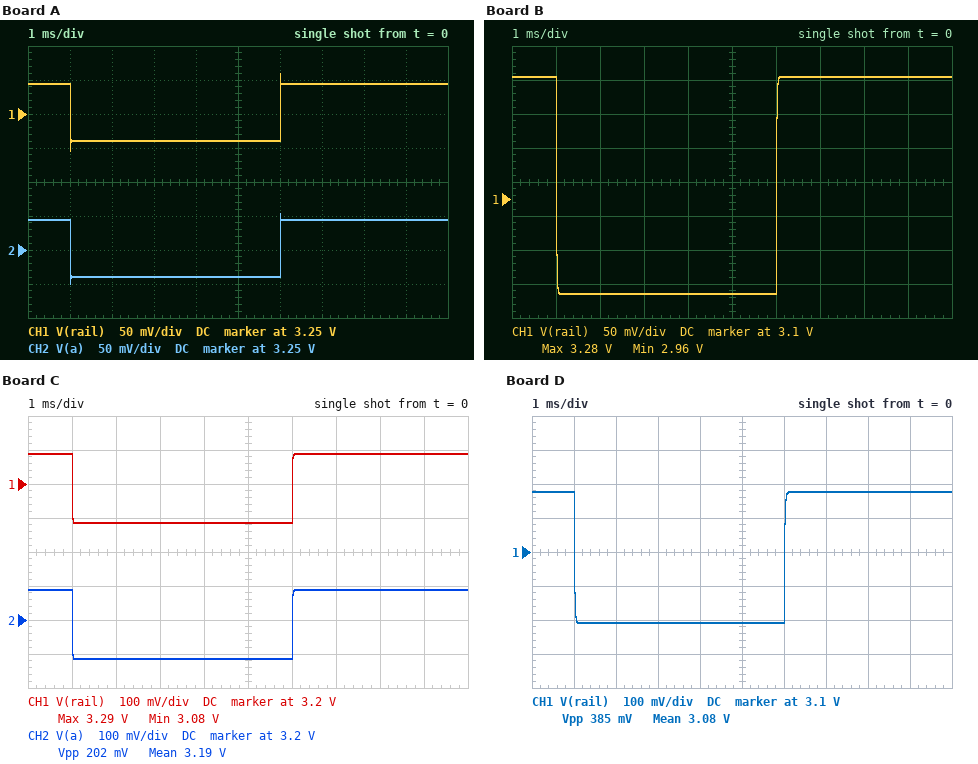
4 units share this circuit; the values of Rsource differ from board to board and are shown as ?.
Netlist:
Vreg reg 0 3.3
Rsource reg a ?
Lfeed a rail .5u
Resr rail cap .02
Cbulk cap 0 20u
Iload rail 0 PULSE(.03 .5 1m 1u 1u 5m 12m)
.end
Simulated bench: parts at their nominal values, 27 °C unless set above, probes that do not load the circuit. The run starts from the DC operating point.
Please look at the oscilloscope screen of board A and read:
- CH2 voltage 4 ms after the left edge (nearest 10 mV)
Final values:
3.21 V
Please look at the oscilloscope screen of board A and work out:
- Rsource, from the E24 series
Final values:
0.18 Ω
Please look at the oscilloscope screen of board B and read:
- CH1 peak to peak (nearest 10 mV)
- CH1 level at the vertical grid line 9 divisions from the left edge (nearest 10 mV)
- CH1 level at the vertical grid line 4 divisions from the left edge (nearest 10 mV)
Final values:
320 mV
3.28 V
2.96 V
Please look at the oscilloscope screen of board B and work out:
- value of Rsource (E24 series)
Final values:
0.68 Ω
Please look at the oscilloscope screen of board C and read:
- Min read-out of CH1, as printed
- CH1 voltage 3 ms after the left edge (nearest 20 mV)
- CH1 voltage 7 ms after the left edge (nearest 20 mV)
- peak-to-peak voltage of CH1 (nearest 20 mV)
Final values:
3.08 V
3.08 V
3.28 V
200 mV
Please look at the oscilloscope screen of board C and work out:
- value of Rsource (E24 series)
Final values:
0.43 Ω
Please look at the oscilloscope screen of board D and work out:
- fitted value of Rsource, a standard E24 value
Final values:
0.82 Ω
